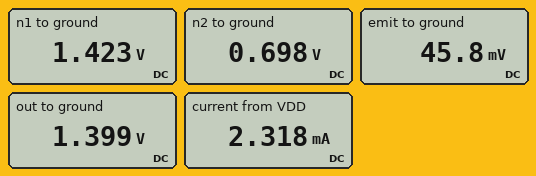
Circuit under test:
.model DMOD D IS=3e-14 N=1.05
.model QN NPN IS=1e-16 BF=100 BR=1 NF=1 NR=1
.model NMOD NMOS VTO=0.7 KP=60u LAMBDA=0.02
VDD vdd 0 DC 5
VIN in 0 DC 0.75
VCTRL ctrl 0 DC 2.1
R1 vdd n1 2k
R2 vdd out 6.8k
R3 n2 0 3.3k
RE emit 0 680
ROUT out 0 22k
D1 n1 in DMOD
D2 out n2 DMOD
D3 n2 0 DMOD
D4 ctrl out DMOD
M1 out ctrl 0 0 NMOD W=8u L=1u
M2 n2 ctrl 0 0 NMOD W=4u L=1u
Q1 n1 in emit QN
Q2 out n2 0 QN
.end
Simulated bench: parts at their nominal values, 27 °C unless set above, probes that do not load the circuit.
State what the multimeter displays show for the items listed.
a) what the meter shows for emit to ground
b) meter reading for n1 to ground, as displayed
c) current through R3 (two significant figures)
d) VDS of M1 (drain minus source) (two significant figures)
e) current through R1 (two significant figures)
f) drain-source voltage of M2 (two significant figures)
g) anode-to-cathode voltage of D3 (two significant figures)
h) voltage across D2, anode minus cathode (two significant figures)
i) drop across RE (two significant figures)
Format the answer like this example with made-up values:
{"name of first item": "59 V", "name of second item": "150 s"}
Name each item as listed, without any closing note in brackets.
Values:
{"what the meter shows for emit to ground": "45.8 mV", "meter reading for n1 to ground, as displayed": "1.423 V", "current through R3": "210 µA", "VDS of M1 (drain minus source)": "1.4 V", "current through R1": "1.8 mA", "drain-source voltage of M2": "700 mV", "anode-to-cathode voltage of D3": "700 mV", "voltage across D2, anode minus cathode": "700 mV", "drop across RE": "46 mV"}
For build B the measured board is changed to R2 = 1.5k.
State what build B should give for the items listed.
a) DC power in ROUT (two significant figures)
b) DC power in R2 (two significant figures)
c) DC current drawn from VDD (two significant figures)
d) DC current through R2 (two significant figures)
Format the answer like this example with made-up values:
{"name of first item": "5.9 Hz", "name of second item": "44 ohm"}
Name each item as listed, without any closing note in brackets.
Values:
{"DC power in ROUT": "90 µW", "DC power in R2": "8.6 mW", "DC current drawn from VDD": "4.2 mA", "DC current through R2": "2.4 mA"}
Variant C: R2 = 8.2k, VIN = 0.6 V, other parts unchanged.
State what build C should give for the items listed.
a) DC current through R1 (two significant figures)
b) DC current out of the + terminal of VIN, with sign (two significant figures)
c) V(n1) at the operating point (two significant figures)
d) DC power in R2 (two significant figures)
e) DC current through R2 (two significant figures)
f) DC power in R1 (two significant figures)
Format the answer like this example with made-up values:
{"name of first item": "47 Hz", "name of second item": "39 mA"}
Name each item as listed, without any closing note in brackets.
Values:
{"DC current through R1": "1.9 mA", "DC current out of the + terminal of VIN, with sign": "-1.9 mA", "V(n1) at the operating point": "1.3 V", "DC power in R2": "1.6 mW", "DC current through R2": "440 µA", "DC power in R1": "6.9 mW"}
